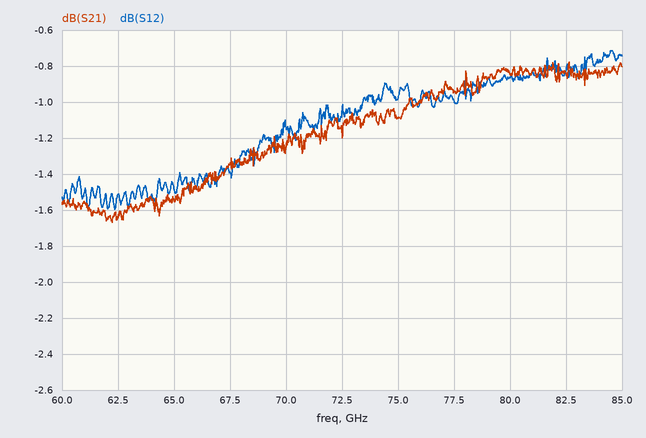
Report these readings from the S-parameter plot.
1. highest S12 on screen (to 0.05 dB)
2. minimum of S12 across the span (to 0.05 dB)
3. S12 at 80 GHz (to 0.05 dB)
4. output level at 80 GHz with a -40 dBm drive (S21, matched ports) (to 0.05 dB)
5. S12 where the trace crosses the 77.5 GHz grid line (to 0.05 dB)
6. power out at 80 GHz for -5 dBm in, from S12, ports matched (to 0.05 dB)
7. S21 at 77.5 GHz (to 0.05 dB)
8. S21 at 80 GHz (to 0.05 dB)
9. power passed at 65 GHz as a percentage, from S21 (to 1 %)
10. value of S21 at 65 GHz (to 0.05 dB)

-0.70 dB
-1.60 dB
-0.85 dB
-40.85 dBm
-1.00 dB
-5.85 dBm
-0.95 dB
-0.85 dB
70 %
-1.55 dB
